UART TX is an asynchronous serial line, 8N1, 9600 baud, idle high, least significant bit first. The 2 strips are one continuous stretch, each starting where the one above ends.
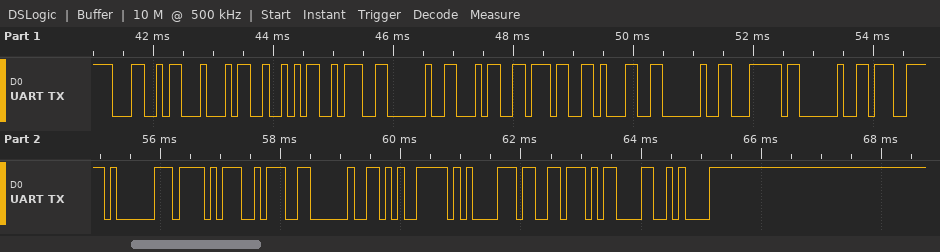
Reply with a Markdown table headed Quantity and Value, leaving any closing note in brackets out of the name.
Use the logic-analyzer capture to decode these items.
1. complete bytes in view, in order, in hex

| Quantity | Value |
|---|---|
| complete bytes in view, in order, in hex | 0x4C 0x44 0x52 0x3A 0x20 0x34 0x37 0x31 0x20 0x7C 0x20 0xE7 0x81 0xAF 0x3A 0x20 0xE5 0x85 0xB3 0x0D 0x0A |
